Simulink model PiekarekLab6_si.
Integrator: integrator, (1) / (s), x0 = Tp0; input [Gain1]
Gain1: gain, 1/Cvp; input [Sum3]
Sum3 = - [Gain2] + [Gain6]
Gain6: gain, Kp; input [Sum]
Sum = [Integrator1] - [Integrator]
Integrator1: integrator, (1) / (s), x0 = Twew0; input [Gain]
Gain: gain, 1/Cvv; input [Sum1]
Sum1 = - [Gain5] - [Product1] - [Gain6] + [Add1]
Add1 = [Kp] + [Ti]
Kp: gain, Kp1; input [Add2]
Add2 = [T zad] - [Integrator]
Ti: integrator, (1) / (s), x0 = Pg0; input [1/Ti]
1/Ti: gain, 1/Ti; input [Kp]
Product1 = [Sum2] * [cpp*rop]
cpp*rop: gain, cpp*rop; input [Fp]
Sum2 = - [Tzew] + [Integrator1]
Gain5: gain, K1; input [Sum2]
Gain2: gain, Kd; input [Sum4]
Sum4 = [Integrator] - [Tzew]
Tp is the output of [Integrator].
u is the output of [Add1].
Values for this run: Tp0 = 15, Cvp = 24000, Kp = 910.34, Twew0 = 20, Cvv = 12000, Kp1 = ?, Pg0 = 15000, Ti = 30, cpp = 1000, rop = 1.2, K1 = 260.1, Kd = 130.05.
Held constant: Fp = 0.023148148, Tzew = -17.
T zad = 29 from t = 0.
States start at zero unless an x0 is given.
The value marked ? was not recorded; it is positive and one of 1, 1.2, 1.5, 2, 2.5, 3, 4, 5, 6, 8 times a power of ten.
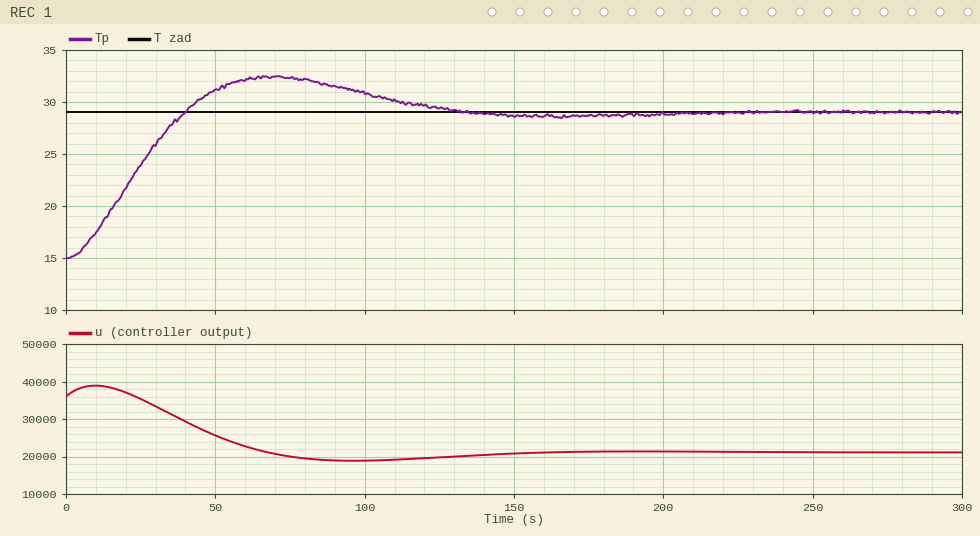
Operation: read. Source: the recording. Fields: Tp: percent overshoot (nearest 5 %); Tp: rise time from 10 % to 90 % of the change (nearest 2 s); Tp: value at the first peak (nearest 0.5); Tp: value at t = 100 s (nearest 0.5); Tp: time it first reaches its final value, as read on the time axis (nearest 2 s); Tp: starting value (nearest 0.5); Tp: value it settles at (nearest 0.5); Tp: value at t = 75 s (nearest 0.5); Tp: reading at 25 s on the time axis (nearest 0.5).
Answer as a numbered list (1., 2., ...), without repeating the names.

1. 25 %
2. 28 s
3. 32.5
4. 31.0
5. 40 s
6. 15.0
7. 29.0
8. 32.5
9. 24.0
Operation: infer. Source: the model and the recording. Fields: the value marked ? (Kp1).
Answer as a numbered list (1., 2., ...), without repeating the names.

1. 1500
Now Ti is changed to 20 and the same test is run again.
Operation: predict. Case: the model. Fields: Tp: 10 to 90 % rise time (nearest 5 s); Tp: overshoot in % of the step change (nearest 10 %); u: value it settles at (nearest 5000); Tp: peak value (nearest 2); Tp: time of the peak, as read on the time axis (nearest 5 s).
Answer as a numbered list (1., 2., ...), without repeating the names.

1. 25 s
2. 40 %
3. 20000
4. 34
5. 60 s
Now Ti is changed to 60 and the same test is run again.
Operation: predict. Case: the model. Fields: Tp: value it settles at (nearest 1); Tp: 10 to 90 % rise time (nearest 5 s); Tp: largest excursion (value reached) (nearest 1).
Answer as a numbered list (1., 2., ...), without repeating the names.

1. 29
2. 35 s
3. 30
